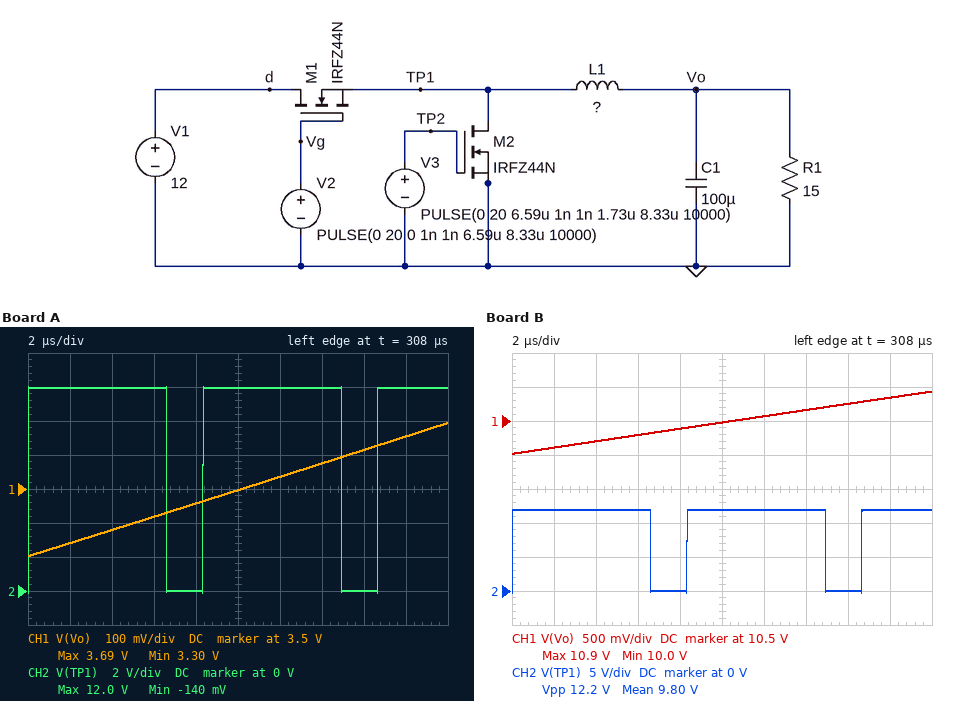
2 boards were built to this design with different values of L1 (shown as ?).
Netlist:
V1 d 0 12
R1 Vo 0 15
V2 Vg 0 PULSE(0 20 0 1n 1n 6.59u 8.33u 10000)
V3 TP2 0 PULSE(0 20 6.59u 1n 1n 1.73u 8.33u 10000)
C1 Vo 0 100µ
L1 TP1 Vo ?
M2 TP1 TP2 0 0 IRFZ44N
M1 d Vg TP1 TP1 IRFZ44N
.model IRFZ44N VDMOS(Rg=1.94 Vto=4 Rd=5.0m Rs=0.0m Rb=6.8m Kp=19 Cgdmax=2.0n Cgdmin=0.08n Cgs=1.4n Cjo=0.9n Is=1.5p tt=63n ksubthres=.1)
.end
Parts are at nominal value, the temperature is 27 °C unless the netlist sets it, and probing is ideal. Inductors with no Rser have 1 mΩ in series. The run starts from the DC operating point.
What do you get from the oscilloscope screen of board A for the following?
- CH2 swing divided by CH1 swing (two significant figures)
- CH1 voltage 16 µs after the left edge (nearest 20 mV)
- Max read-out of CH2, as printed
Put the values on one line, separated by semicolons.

31; 3.62 V; 12.0 V
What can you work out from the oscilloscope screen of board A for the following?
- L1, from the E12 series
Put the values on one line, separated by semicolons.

1.2 mH
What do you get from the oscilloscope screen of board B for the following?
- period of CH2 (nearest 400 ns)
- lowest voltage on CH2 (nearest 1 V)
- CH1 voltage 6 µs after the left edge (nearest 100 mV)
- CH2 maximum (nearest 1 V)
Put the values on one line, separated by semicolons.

8.4 µs; 0 V; 10.3 V; 12 V
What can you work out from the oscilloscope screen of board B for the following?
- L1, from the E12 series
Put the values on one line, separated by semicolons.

330 µH
